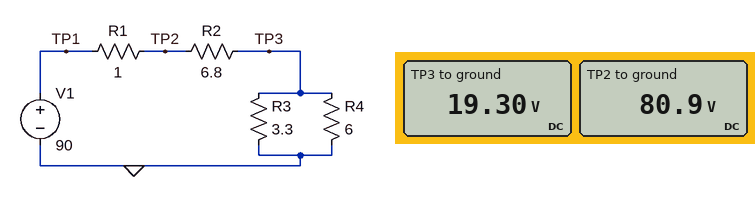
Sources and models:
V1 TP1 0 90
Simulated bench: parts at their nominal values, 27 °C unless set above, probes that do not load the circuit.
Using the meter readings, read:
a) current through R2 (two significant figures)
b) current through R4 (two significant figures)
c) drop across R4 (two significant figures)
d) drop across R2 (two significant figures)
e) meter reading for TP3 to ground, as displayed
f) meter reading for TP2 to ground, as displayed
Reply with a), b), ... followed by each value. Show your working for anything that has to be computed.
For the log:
a) (80.9 V - 19.3 V) / 6.8 Ω = 9.1 A
b) (19.3 V) / 6 Ω = 3.2 A
c) 19.3 V = 19 V
d) 80.9 V - 19.3 V = 62 V
e) 19.30 V
f) 80.9 V
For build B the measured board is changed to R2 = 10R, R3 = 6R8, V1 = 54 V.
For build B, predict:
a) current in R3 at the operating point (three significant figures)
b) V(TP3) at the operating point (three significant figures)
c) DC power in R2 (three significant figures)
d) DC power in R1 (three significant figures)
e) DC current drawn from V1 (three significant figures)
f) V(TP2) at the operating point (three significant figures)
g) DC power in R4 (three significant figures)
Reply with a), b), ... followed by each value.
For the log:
a) 1.78 A
b) 12.1 V
c) 145 W
d) 14.5 W
e) 3.81 A
f) 50.2 V
g) 24.5 W
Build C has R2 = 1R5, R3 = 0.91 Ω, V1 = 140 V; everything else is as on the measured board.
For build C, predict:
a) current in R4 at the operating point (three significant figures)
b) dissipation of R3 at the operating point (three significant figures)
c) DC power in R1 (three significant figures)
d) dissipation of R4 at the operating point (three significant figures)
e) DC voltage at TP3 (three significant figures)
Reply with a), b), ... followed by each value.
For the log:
a) 5.60 A
b) 1.24 kW
c) 1.81 kW
d) 188 W
e) 33.6 V
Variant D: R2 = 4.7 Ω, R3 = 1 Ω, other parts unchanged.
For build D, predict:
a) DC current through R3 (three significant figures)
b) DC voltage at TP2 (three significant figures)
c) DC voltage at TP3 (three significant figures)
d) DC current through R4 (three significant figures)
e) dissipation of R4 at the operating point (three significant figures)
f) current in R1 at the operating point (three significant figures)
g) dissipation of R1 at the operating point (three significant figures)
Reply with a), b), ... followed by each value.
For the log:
a) 11.8 A
b) 76.3 V
c) 11.8 V
d) 1.96 A
e) 23.1 W
f) 13.7 A
g) 188 W
